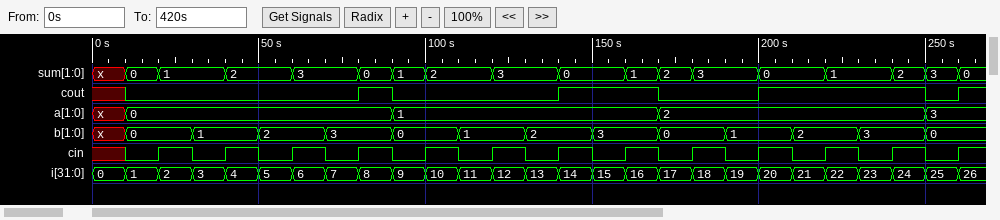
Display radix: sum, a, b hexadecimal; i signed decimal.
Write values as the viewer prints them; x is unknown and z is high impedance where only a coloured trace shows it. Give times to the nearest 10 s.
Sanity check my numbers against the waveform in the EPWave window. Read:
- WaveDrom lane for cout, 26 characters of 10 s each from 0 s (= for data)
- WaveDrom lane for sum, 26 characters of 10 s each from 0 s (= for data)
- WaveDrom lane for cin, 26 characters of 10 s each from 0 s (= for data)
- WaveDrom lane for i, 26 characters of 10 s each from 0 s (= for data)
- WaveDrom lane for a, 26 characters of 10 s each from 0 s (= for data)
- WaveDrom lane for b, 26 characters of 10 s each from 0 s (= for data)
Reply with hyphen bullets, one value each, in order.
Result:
- {name: 'cout', wave: 'x0......10....1..0..1....0'}
- {name: 'sum', wave: 'x==.=.=.===.=.=.===.=.=.==', data: '0 1 2 3 0 1 2 3 0 1 2 3 0 1 2 3'}
- {name: 'cin', wave: 'x0101010101010101010101010'}
- {name: 'i', wave: '==========================', data: '0 1 2 3 4 5 6 7 8 9 10 11 12 13 14 15 16 17 18 19 20 21 22 23 24 25'}
- {name: 'a', wave: 'x=.......=.......=.......=', data: '0 1 2 3'}
- {name: 'b', wave: 'x=.=.=.=.=.=.=.=.=.=.=.=.=', data: '0 1 2 3 0 1 2 3 0 1 2 3 0'}
